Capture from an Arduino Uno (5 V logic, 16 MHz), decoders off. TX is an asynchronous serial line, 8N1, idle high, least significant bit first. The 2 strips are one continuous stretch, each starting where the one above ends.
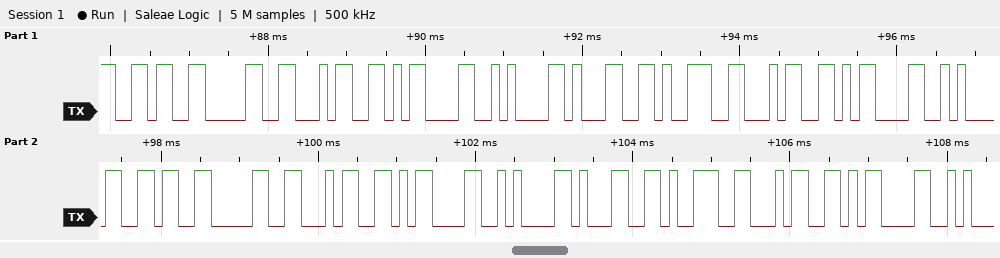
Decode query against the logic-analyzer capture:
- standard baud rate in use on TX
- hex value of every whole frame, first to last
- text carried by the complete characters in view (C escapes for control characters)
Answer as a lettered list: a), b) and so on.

a) 9600 baud
b) 36 30 34 0D 0A 31 39 34 0D 0A 36 30 34 0D 0A 31 39 34 0D
c) "604\r\n194\r\n604\r\n194\r"
